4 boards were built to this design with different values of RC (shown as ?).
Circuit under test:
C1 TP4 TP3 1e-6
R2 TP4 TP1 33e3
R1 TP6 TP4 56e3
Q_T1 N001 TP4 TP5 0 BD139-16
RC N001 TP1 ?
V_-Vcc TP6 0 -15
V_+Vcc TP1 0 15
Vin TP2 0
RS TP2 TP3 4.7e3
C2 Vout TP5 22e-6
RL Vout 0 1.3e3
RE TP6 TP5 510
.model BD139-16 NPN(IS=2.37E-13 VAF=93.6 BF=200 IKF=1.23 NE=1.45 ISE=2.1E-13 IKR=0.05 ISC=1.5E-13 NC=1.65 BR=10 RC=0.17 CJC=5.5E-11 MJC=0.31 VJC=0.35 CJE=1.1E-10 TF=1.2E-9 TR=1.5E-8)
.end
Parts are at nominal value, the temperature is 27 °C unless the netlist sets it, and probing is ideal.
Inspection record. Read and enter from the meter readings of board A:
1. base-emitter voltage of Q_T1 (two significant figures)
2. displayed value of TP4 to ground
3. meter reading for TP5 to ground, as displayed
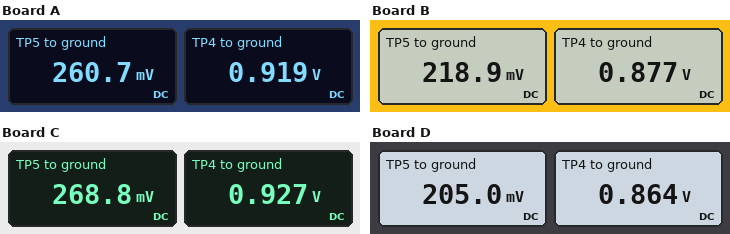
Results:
660 mV
0.919 V
260.7 mV
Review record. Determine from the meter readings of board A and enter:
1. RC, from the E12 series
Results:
39 Ω
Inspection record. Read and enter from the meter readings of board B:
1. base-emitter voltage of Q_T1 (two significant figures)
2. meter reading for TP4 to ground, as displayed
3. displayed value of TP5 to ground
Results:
660 mV
0.877 V
218.9 mV
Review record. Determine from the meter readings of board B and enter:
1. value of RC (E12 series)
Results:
100 Ω
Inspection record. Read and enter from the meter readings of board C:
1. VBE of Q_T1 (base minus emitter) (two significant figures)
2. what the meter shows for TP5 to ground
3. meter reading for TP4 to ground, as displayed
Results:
660 mV
268.8 mV
0.927 V
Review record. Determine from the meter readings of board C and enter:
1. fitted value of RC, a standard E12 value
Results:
27 Ω
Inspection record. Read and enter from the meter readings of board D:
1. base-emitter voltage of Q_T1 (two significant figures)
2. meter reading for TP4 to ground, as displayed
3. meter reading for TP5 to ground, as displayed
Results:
660 mV
0.864 V
205.0 mV
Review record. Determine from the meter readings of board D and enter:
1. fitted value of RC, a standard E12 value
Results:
120 Ω
